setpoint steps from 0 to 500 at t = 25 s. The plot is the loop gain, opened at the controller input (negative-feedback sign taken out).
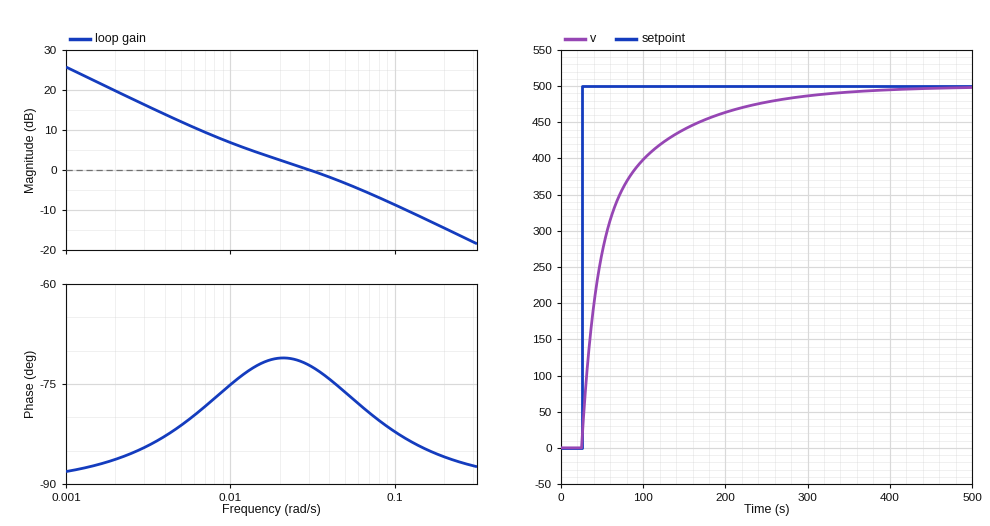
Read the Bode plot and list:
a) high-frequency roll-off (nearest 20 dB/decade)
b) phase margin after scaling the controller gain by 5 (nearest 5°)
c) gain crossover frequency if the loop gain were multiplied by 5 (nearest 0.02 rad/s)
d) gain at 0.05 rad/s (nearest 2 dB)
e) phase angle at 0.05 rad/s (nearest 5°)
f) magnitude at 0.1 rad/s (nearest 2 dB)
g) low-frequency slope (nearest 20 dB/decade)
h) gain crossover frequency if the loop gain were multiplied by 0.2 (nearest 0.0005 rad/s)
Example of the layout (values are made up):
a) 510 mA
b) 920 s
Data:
a) -20 dB/decade
b) 95°
c) 0.18 rad/s
d) -4 dB
e) -75°
f) -8 dB
g) -20 dB/decade
h) 0.0040 rad/s
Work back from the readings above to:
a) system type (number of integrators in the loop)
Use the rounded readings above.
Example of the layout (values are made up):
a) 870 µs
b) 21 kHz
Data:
a) 1
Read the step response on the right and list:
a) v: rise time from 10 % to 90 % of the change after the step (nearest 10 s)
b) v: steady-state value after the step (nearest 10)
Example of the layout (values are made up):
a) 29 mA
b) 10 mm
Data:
a) 140 s
b) 500
